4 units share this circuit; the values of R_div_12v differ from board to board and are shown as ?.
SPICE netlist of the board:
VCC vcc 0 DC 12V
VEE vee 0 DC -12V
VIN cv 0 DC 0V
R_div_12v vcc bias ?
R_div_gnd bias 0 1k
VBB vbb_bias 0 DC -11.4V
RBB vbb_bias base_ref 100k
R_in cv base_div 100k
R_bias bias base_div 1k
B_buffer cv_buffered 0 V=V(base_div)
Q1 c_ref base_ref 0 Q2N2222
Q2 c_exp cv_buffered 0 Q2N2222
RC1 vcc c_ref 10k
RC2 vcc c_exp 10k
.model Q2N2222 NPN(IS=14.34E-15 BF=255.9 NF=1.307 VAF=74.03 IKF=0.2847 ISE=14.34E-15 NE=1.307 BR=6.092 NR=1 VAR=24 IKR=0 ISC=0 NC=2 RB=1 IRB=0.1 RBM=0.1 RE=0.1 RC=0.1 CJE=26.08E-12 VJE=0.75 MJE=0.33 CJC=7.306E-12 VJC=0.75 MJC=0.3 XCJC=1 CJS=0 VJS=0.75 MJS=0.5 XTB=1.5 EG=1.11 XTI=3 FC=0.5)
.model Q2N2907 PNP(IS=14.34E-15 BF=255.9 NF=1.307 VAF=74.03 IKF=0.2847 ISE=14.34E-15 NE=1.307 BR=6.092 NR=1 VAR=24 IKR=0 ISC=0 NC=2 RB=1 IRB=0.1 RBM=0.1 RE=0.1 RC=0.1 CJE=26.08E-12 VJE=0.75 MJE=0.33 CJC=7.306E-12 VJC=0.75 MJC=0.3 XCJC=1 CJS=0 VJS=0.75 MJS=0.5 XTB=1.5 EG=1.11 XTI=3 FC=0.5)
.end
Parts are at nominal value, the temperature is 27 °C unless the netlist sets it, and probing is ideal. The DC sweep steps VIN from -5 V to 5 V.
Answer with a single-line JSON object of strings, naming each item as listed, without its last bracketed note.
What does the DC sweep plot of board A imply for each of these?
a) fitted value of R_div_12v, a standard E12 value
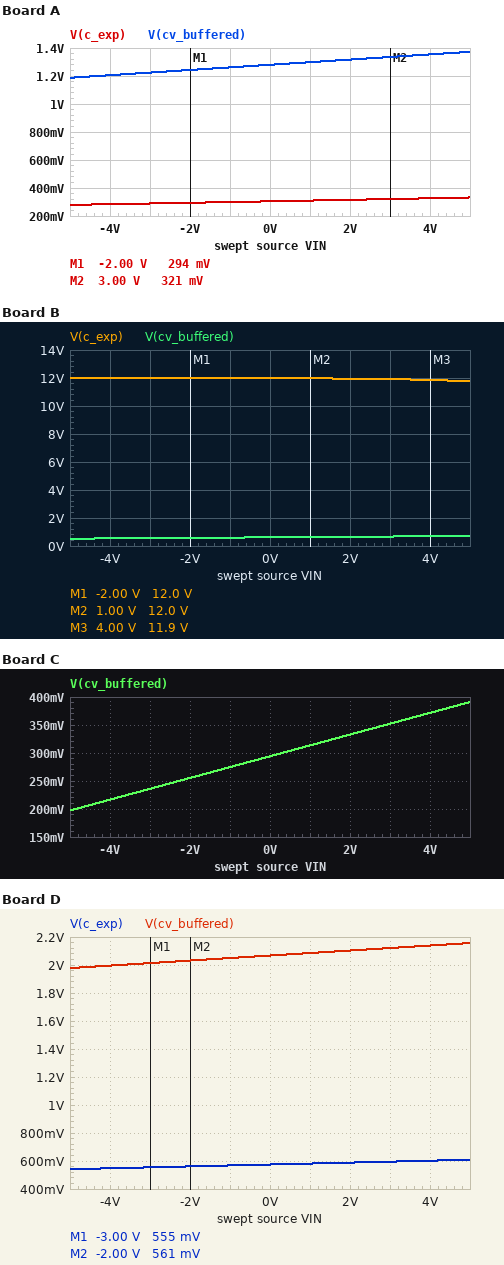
{"fitted value of R_div_12v, a standard E12 value": "8.2 kΩ"}
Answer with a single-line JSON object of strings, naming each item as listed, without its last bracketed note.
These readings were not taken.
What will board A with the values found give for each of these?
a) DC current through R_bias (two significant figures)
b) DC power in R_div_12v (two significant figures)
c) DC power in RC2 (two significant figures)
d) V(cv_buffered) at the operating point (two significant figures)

{"DC current through R_bias": "13 µA", "DC power in R_div_12v": "14 mW", "DC power in RC2": "14 mW", "V(cv_buffered) at the operating point": "1.3 V"}
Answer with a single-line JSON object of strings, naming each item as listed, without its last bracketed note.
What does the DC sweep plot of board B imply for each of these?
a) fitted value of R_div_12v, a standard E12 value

{"fitted value of R_div_12v, a standard E12 value": "18 kΩ"}
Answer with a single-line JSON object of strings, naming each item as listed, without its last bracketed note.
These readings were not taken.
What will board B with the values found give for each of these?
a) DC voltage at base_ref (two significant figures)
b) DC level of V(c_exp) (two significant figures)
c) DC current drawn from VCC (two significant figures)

{"DC voltage at base_ref": "-11 V", "DC level of V(c_exp)": "12 V", "DC current drawn from VCC": "630 µA"}
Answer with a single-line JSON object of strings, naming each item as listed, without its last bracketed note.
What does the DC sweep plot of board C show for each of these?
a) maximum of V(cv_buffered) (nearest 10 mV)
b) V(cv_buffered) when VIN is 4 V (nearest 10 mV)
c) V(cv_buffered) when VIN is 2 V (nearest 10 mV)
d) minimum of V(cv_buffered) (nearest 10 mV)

{"maximum of V(cv_buffered)": "390 mV", "V(cv_buffered) when VIN is 4 V": "370 mV", "V(cv_buffered) when VIN is 2 V": "330 mV", "minimum of V(cv_buffered)": "200 mV"}
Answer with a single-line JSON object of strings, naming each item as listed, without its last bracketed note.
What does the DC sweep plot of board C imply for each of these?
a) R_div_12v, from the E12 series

{"R_div_12v, from the E12 series": "39 kΩ"}
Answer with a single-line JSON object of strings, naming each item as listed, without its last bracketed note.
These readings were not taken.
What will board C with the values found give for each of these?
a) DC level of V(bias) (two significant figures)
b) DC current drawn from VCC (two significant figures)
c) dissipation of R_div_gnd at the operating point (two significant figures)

{"DC level of V(bias)": "300 mV", "DC current drawn from VCC": "300 µA", "dissipation of R_div_gnd at the operating point": "88 µW"}
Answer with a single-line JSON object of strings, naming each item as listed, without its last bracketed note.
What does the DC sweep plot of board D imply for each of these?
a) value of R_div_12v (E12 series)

{"value of R_div_12v": "4.7 kΩ"}
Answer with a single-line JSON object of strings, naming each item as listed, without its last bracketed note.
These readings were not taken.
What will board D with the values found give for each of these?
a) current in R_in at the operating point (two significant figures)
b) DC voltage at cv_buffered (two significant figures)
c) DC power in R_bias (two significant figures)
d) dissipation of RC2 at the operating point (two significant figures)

{"current in R_in at the operating point": "21 µA", "DC voltage at cv_buffered": "2.1 V", "DC power in R_bias": "430 nW", "dissipation of RC2 at the operating point": "13 mW"}
